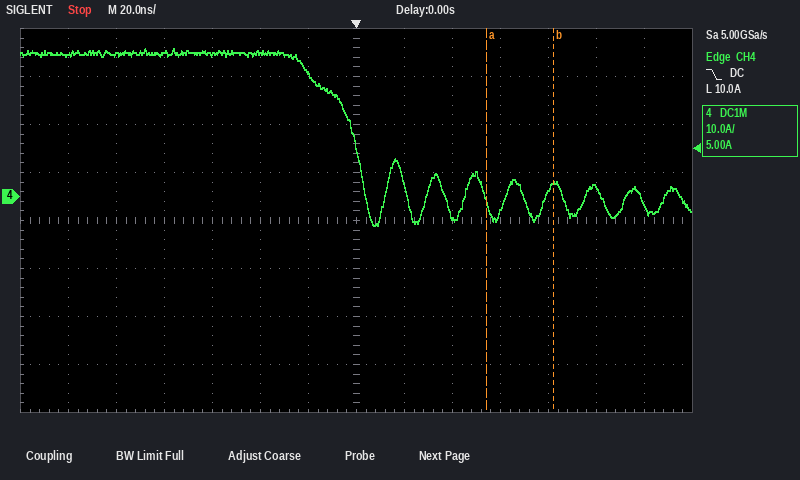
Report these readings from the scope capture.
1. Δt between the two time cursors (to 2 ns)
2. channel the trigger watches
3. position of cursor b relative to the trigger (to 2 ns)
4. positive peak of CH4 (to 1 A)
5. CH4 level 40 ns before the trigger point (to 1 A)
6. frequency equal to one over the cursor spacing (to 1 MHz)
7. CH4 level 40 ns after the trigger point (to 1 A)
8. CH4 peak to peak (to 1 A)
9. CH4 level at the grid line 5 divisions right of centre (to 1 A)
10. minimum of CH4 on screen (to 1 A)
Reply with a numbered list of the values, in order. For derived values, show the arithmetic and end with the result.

1. 28 ns
2. CH4
3. +82 ns
4. 31 A
5. 30 A
6. 1 / 28 ns ≈ 36 MHz
7. -4 A
8. 31 A − (-6 A) = 37 A
9. 2 A
10. -6 A
